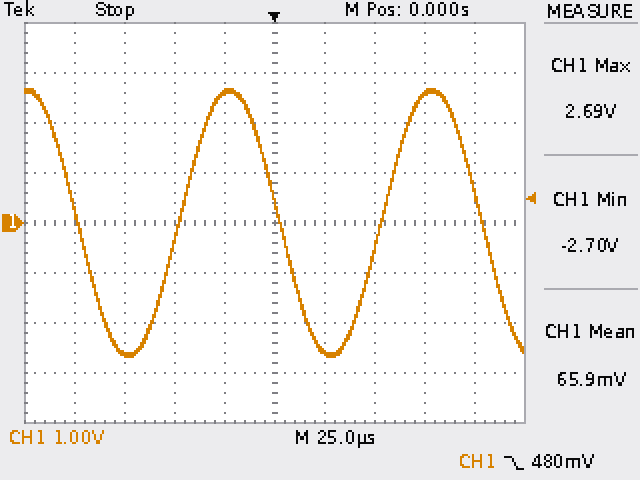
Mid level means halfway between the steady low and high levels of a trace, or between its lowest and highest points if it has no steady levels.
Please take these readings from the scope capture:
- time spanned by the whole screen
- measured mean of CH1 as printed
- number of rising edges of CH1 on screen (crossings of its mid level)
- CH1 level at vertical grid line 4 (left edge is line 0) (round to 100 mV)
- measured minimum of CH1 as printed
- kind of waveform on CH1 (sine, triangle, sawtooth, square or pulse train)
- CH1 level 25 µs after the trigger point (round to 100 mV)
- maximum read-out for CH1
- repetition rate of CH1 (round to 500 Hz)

250 µs
65.9 mV
2
2.6 V
-2.70 V
sine
-2.6 V
2.69 V
10.0 kHz
